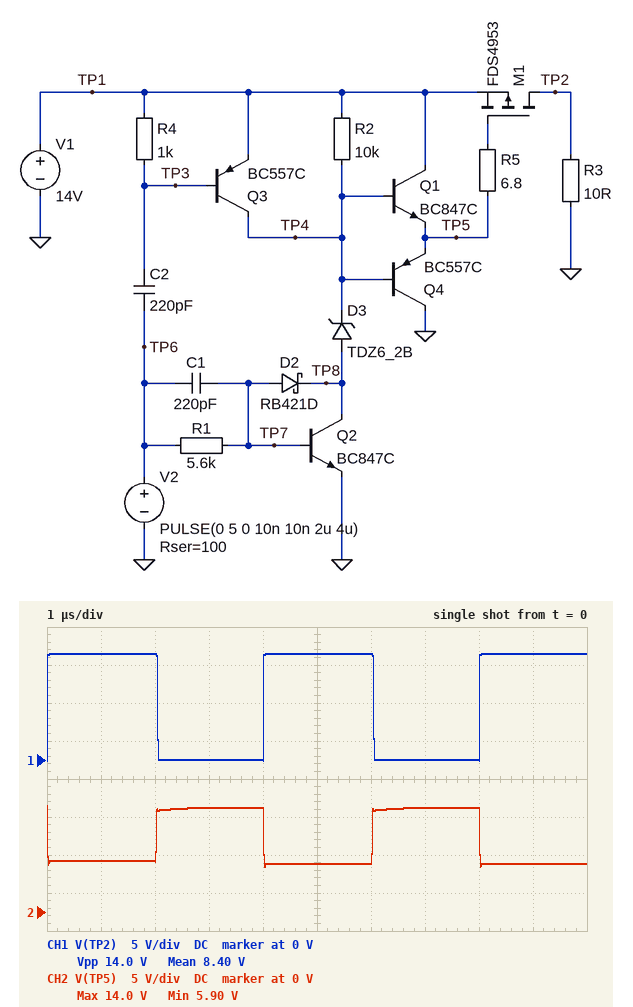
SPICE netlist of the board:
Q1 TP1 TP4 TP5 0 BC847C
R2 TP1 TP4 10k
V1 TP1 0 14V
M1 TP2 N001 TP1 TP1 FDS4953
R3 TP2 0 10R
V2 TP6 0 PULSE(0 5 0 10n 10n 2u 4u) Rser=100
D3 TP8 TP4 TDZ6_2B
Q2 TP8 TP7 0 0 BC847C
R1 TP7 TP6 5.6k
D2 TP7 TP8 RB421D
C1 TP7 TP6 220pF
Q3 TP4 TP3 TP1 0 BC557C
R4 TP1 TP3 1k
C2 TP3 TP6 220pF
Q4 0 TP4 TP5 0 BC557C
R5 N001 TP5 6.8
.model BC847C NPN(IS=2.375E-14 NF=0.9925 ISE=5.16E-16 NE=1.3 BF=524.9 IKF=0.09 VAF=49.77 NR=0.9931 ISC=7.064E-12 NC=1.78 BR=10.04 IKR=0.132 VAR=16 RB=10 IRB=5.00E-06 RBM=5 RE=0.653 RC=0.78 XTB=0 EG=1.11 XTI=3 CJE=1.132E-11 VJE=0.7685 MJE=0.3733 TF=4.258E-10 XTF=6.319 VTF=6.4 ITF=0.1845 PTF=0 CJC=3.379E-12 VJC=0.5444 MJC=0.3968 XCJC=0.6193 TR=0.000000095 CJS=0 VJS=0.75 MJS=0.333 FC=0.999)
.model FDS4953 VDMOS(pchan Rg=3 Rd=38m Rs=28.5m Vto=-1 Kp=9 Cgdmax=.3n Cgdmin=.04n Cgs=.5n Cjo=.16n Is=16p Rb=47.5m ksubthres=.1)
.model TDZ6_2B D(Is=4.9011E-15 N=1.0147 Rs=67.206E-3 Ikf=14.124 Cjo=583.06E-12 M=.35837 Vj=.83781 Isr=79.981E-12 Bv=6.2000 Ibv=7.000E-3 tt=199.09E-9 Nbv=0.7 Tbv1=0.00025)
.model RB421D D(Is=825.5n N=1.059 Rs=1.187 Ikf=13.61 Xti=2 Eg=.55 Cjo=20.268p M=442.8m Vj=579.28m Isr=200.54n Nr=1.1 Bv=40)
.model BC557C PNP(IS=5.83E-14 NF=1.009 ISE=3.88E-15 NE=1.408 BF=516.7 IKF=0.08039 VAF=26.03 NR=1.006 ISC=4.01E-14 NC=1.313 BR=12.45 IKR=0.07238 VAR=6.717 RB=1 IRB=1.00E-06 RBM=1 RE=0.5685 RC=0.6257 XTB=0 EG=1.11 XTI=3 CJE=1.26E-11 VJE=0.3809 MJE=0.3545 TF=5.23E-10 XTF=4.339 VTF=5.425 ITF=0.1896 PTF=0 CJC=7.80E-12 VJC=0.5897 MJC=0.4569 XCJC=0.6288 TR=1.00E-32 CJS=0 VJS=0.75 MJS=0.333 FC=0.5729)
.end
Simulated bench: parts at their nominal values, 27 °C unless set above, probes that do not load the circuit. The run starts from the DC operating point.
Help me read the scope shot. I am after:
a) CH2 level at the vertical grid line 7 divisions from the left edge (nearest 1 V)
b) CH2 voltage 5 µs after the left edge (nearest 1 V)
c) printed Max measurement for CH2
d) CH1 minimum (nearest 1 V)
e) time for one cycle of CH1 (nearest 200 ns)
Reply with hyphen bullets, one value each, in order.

- 14 V
- 6 V
- 14.0 V
- 0 V
- 4.0 µs
